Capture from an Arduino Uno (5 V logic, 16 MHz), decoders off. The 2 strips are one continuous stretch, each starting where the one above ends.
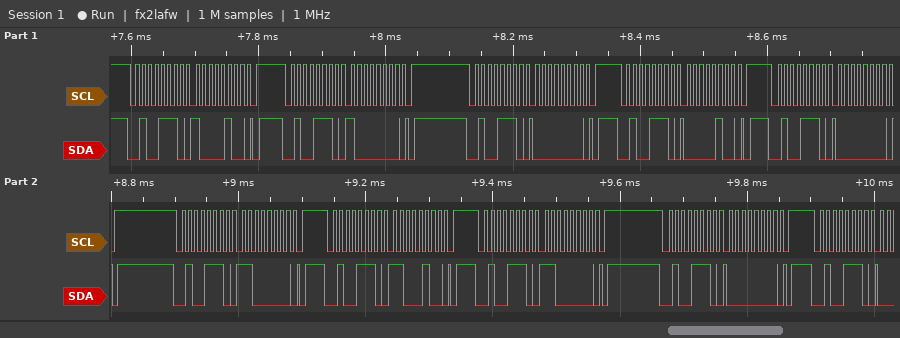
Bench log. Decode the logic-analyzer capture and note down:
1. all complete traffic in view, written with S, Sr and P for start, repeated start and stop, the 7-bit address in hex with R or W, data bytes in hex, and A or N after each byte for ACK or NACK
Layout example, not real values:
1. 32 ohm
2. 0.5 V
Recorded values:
1. S 27W A 84 A P S 27W A 80 A P S 27W A 00 A P S 27W A 04 A P S 27W A 00 A P S 27W A C0 A P S 27W A C4 A P S 27W A C0 A P S 27W A 00 A P S 27W A
